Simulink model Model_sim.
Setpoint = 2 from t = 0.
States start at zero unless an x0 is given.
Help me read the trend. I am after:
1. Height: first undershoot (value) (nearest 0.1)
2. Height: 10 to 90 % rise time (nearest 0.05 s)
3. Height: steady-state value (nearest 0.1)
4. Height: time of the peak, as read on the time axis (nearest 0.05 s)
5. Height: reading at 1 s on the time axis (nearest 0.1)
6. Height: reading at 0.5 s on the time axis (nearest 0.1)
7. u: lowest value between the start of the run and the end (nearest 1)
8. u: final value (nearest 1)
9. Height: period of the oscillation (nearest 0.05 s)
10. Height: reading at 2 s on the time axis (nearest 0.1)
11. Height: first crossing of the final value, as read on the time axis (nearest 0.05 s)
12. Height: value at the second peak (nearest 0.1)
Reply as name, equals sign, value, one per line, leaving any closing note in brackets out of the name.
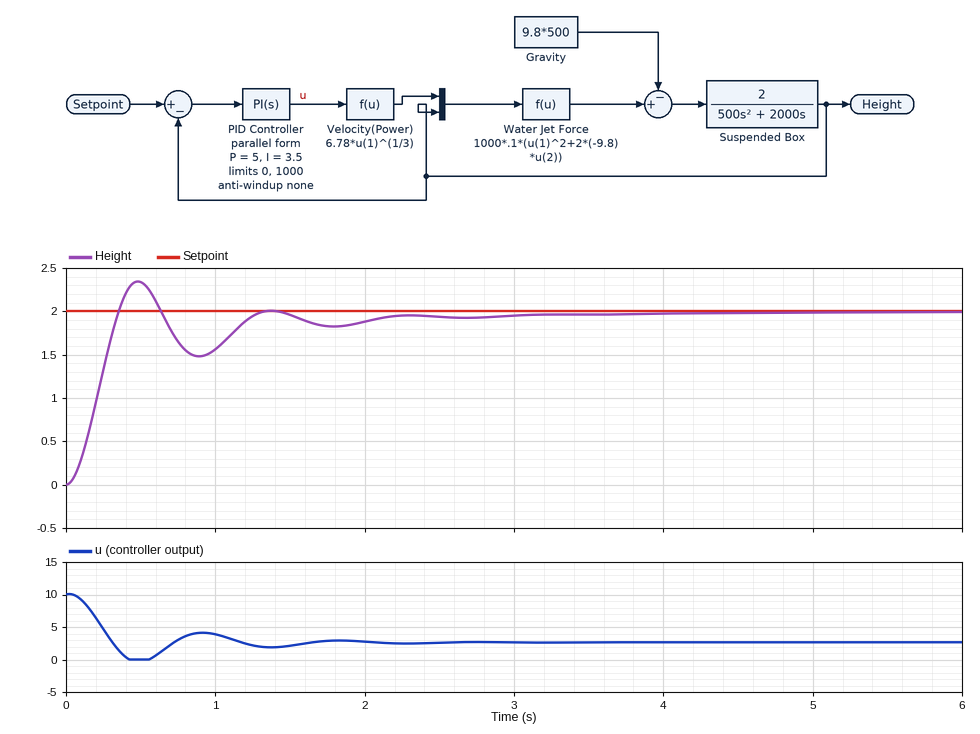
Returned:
Height: first undershoot (value) = 1.5
Height: 10 to 90 % rise time = 0.25 s
Height: steady-state value = 2.0
Height: time of the peak, as read on the time axis = 0.50 s
Height: reading at 1 s on the time axis = 1.6
Height: reading at 0.5 s on the time axis = 2.3
u: lowest value between the start of the run and the end = 0
u: final value = 3
Height: period of the oscillation = 0.90 s
Height: reading at 2 s on the time axis = 1.9
Height: first crossing of the final value, as read on the time axis = 0.35 s
Height: value at the second peak = 2.0
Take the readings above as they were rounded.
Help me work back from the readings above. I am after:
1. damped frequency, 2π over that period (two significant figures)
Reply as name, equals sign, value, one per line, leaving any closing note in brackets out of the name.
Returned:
damped frequency, 2π over that period = 7.0 rad/s
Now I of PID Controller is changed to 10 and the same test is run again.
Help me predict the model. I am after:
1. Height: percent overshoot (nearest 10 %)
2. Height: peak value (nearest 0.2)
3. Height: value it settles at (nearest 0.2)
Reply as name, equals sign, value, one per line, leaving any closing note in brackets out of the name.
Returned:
Height: percent overshoot = 40 %
Height: peak value = 2.8
Height: value it settles at = 2.0
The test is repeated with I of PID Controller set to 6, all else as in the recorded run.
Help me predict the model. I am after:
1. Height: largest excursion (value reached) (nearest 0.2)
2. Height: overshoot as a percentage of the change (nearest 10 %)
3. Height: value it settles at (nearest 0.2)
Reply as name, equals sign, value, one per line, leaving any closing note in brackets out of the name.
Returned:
Height: largest excursion (value reached) = 2.6
Height: overshoot as a percentage of the change = 30 %
Height: value it settles at = 2.0
